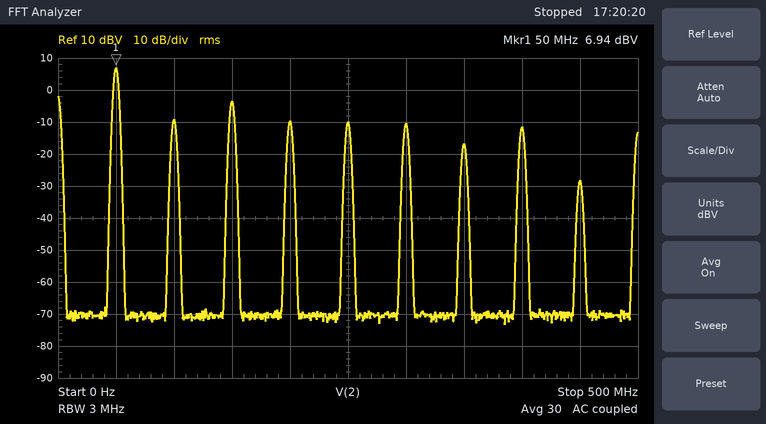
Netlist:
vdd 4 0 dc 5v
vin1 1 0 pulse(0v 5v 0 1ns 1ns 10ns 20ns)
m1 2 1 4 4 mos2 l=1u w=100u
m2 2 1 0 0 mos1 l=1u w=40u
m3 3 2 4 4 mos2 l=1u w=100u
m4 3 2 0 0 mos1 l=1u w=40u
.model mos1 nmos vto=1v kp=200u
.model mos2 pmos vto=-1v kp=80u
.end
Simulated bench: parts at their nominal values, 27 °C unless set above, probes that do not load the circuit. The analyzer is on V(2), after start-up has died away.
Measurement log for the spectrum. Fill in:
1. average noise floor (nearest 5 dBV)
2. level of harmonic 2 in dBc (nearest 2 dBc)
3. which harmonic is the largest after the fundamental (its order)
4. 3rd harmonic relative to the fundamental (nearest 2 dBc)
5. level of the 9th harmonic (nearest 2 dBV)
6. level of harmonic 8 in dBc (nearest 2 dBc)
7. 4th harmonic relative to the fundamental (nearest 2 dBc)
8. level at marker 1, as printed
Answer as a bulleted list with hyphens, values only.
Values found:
- -70 dBV
- -16 dBc
- 3
- -10 dBc
- -28 dBV
- -18 dBc
- -16 dBc
- 6.94 dBV
